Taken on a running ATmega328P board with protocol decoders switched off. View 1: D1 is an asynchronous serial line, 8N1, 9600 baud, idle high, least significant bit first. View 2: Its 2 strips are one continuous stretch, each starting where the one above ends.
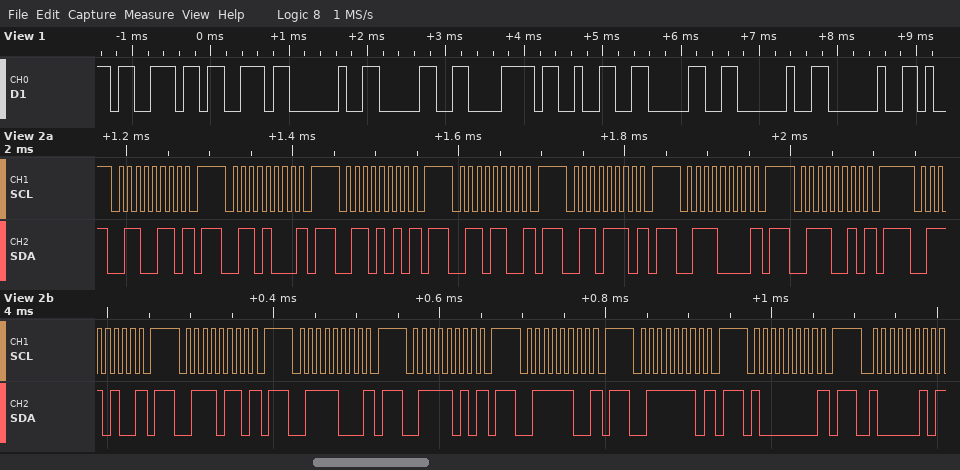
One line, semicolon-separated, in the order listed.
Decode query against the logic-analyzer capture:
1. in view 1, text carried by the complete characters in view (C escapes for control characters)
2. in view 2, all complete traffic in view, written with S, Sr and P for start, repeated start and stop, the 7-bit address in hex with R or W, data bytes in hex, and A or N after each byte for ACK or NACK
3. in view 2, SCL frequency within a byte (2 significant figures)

"ss 0x20  "; S 33W N P S 34W N P S 35W N P S 36W N P S 37W N P S 38W N P S 39W N P S 3AW N P S 3BW N P S 3CW N P S 3DW N P S 3EW N P S 3FW N P S 40W N P S 41W N; 100 kHz
